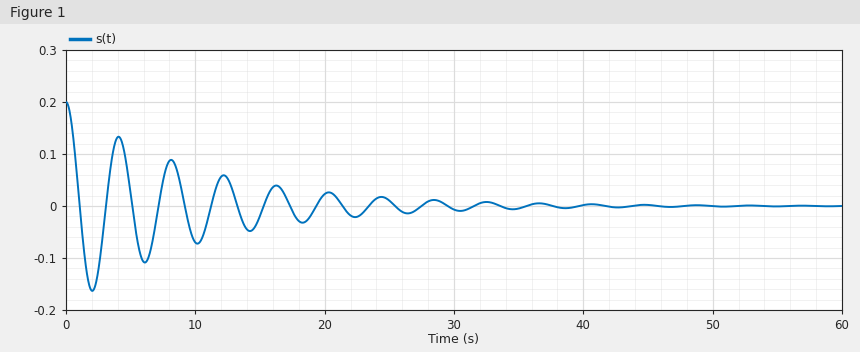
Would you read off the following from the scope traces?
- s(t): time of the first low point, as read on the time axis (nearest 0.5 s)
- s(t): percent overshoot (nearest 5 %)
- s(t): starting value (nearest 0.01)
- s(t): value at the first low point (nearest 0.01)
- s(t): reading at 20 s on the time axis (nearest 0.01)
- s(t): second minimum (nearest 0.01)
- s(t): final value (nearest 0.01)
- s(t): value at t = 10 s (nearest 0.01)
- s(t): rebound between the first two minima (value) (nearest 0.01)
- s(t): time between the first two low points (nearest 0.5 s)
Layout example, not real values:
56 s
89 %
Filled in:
2.0 s
80 %
0.20
-0.16
0.02
-0.11
0.00
-0.07
0.13
4.0 s
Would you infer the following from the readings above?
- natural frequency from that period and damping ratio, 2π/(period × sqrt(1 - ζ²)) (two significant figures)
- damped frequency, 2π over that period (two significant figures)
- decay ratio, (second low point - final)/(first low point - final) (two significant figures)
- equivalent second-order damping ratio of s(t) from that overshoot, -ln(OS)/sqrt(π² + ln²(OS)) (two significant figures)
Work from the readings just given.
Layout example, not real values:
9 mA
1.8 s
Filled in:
1.6 rad/s
1.6 rad/s
0.69
0.071
